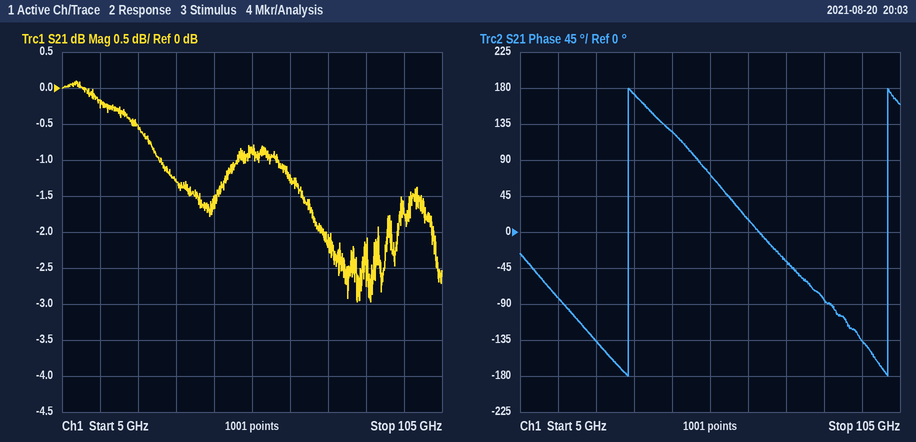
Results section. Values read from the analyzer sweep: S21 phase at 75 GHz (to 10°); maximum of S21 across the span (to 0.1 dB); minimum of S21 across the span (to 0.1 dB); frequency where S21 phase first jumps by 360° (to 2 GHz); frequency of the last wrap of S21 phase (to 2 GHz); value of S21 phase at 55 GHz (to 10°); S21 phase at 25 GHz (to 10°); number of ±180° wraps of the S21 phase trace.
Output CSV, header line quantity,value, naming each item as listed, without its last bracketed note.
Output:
quantity,value
S21 phase at 75 GHz,-40°
maximum of S21 across the span,0.1 dB
minimum of S21 across the span,-3.0 dB
frequency where S21 phase first jumps by 360°,34 GHz
frequency of the last wrap of S21 phase,102 GHz
value of S21 phase at 55 GHz,70°
S21 phase at 25 GHz,-140°
number of ±180° wraps of the S21 phase trace,2
